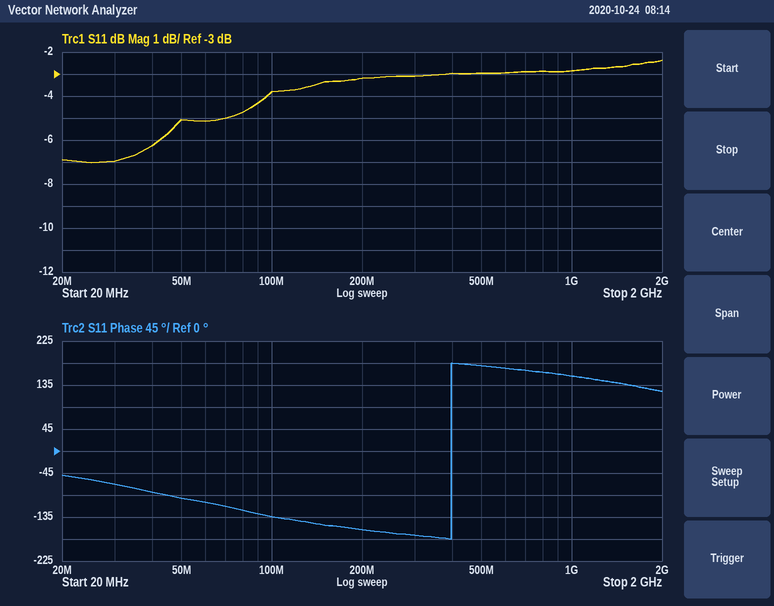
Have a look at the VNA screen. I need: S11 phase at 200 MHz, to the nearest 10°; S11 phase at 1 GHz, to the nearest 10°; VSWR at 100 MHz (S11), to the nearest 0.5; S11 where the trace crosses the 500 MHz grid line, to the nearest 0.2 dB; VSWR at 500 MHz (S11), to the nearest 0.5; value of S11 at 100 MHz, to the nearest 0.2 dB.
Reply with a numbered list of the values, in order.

1. -160°
2. 150°
3. 4.5
4. -3.0 dB
5. 6.0
6. -3.8 dB
